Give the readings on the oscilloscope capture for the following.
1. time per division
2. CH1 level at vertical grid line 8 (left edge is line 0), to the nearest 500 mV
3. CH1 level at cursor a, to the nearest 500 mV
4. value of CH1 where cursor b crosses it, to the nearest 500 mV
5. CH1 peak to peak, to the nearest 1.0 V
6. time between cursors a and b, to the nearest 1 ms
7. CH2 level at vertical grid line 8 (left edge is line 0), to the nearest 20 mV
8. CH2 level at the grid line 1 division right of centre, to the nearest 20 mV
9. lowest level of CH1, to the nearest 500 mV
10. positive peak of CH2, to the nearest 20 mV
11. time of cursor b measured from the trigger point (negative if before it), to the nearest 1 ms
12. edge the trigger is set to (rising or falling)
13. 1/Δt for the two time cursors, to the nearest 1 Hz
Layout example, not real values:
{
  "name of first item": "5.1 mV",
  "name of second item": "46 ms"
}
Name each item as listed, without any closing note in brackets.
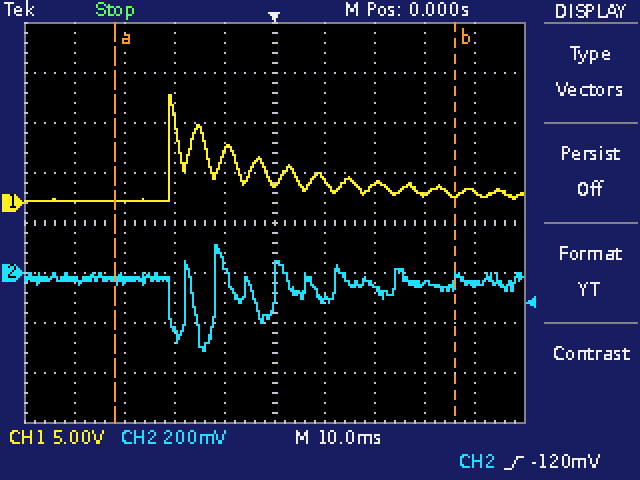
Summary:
{
  "time per division": "10 ms",
  "CH1 level at vertical grid line 8 (left edge is line 0), to the nearest 500 mV": "1.0 V",
  "CH1 level at cursor a, to the nearest 500 mV": "0.0 V",
  "value of CH1 where cursor b crosses it, to the nearest 500 mV": "1.0 V",
  "CH1 peak to peak, to the nearest 1.0 V": "11.0 V",
  "time between cursors a and b, to the nearest 1 ms": "68 ms",
  "CH2 level at vertical grid line 8 (left edge is line 0), to the nearest 20 mV": "-40 mV",
  "CH2 level at the grid line 1 division right of centre, to the nearest 20 mV": "-100 mV",
  "lowest level of CH1, to the nearest 500 mV": "0.0 V",
  "positive peak of CH2, to the nearest 20 mV": "120 mV",
  "time of cursor b measured from the trigger point (negative if before it), to the nearest 1 ms": "+36 ms",
  "edge the trigger is set to": "rising",
  "1/Δt for the two time cursors, to the nearest 1 Hz": "15 Hz"
}
